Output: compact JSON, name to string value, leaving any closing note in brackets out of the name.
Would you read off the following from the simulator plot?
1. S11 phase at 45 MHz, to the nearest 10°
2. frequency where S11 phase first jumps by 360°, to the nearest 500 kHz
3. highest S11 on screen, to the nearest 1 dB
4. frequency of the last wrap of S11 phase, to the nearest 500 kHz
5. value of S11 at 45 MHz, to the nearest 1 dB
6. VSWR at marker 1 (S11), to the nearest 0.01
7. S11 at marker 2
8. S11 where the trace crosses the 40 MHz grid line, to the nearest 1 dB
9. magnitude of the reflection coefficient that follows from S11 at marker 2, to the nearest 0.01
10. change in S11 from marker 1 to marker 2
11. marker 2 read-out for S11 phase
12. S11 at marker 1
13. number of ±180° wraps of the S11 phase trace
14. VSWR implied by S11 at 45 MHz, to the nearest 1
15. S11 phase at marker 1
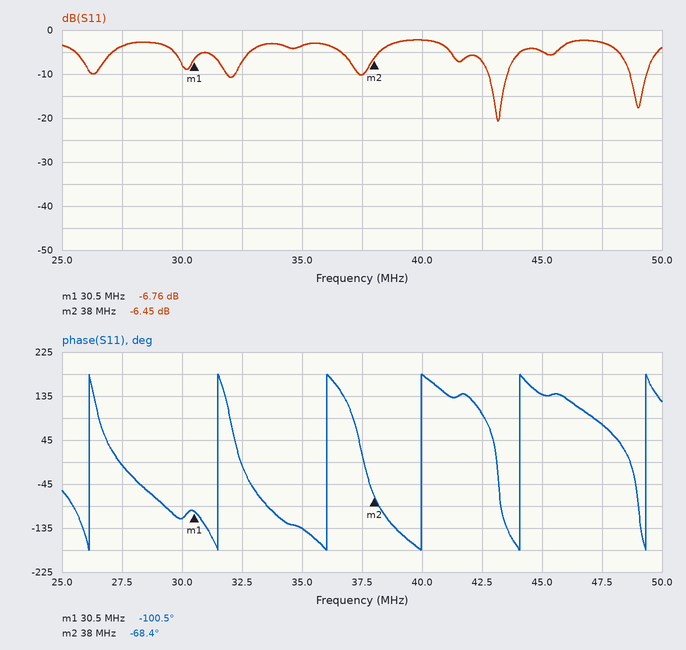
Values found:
{"S11 phase at 45 MHz, to the nearest 10°": "140°", "frequency where S11 phase first jumps by 360°, to the nearest 500 kHz": "26.0 MHz", "highest S11 on screen, to the nearest 1 dB": "-2 dB", "frequency of the last wrap of S11 phase, to the nearest 500 kHz": "49.5 MHz", "value of S11 at 45 MHz, to the nearest 1 dB": "-5 dB", "VSWR at marker 1 (S11), to the nearest 0.01": "2.70", "S11 at marker 2": "-6.45 dB", "S11 where the trace crosses the 40 MHz grid line, to the nearest 1 dB": "-2 dB", "magnitude of the reflection coefficient that follows from S11 at marker 2, to the nearest 0.01": "0.48", "change in S11 from marker 1 to marker 2": "0.31 dB", "marker 2 read-out for S11 phase": "-68.4°", "S11 at marker 1": "-6.76 dB", "number of ±180° wraps of the S11 phase trace": "6", "VSWR implied by S11 at 45 MHz, to the nearest 1": "4", "S11 phase at marker 1": "-100.5°"}
